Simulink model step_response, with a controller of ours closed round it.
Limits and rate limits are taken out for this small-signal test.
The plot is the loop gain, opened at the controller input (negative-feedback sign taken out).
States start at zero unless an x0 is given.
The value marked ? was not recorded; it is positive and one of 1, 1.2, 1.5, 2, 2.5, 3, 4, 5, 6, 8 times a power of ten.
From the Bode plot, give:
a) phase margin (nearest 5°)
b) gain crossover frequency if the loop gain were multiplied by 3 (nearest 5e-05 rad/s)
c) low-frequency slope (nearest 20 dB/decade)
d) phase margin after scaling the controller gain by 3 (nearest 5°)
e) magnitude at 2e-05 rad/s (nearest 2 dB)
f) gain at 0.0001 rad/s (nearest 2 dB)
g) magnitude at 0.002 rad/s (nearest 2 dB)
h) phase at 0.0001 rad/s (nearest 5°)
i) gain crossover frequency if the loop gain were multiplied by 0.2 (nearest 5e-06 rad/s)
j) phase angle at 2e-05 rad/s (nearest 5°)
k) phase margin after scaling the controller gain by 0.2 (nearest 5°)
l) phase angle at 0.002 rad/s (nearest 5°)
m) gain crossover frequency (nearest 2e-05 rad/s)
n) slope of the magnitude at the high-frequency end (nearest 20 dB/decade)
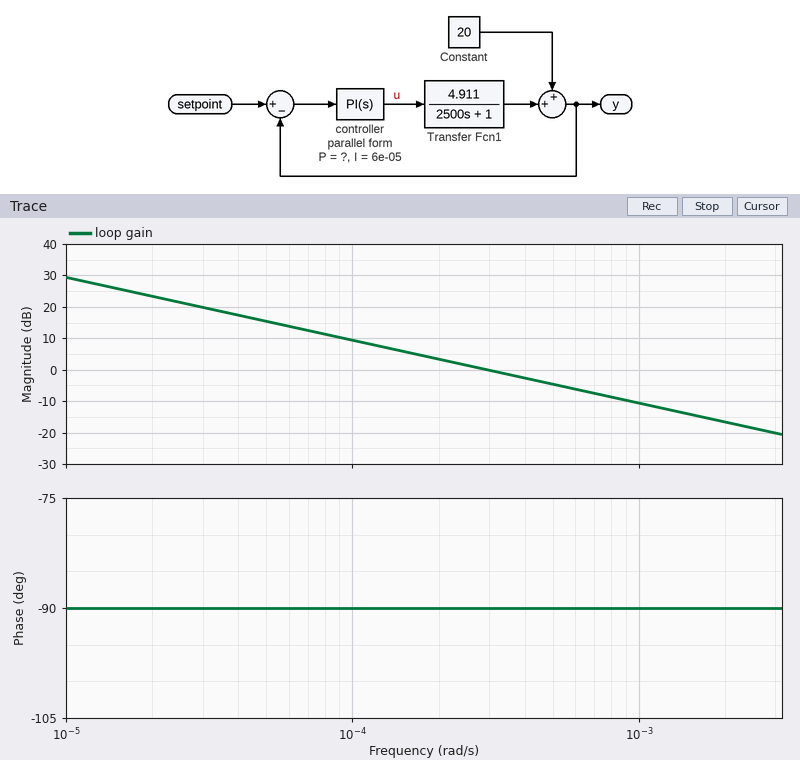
90°
0.00090 rad/s
-20 dB/decade
90°
24 dB
10 dB
-16 dB
-90°
0.000060 rad/s
-90°
90°
-90°
0.00030 rad/s
-20 dB/decade
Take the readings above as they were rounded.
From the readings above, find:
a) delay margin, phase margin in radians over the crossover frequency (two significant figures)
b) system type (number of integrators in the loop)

5200 s
1
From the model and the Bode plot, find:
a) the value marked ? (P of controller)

0.15
